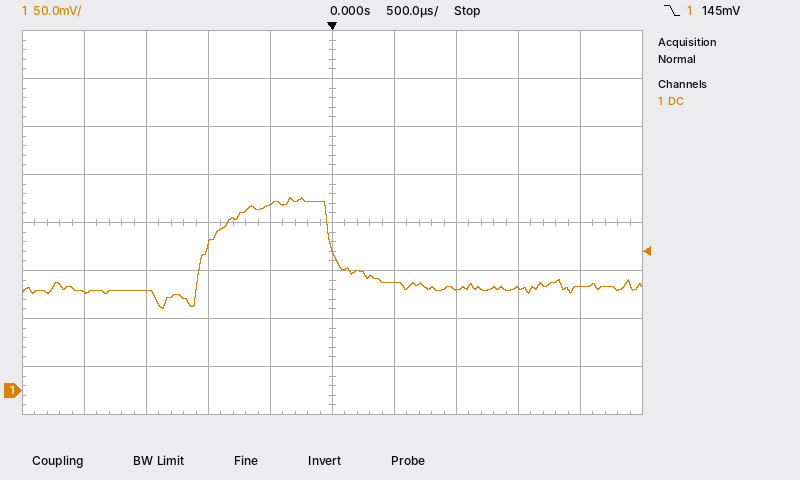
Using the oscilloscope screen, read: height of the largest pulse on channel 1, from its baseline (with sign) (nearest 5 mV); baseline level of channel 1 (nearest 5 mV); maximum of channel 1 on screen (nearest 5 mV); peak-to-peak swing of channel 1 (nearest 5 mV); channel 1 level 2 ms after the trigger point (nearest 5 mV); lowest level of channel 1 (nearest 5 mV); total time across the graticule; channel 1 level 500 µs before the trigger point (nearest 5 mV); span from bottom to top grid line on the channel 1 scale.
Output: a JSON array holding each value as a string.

["+95 mV", "105 mV", "200 mV", "115 mV", "110 mV", "85 mV", "5 ms", "195 mV", "400 mV"]
